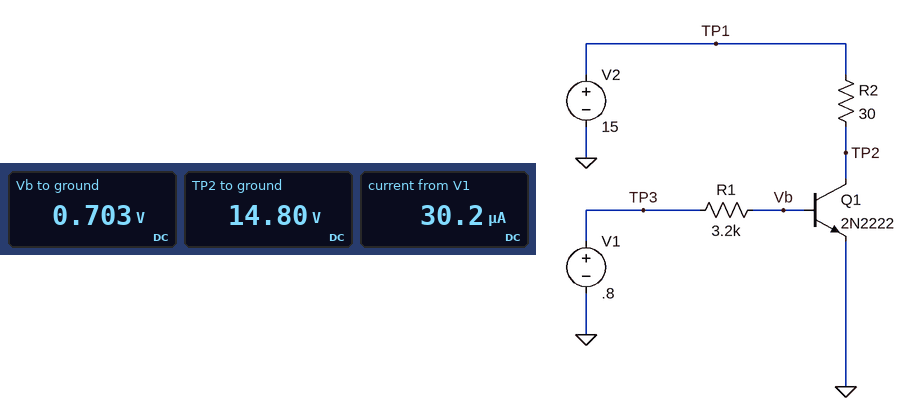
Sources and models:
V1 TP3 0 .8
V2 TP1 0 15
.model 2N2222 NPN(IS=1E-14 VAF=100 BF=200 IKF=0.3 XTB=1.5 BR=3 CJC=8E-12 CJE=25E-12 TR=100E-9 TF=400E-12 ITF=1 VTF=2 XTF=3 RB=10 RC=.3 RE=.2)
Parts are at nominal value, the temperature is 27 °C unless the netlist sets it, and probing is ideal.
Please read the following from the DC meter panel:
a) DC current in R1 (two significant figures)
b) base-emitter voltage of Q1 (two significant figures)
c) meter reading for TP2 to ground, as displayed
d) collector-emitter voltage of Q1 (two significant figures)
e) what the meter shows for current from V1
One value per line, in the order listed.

30 µA
700 mV
14.80 V
15 V
30.2 µA
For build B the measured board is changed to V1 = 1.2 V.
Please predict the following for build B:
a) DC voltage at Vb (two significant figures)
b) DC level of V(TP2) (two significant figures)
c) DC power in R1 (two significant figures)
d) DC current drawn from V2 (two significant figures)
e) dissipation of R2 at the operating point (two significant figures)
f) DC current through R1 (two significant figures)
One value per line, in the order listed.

750 mV
14 V
64 µW
29 mA
26 mW
140 µA
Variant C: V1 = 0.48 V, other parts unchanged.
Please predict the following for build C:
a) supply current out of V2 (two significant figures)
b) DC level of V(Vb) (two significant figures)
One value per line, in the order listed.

1.3 µA
480 mV
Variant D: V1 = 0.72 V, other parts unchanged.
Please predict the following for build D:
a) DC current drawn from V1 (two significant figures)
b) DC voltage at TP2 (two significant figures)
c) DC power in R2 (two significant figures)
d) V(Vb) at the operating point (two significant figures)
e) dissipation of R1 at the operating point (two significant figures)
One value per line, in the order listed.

13 µA
15 V
240 µW
680 mV
510 nW
